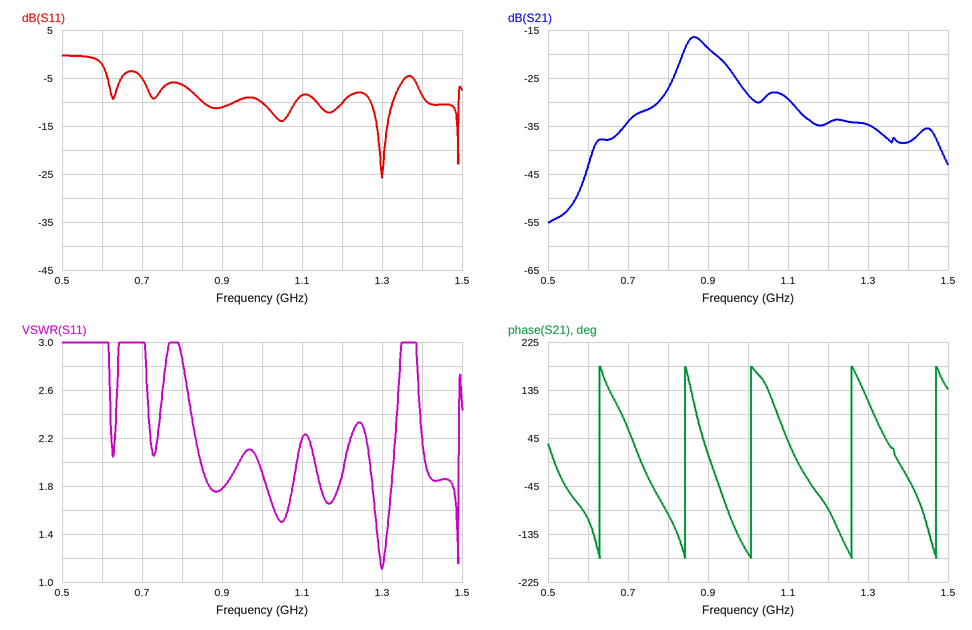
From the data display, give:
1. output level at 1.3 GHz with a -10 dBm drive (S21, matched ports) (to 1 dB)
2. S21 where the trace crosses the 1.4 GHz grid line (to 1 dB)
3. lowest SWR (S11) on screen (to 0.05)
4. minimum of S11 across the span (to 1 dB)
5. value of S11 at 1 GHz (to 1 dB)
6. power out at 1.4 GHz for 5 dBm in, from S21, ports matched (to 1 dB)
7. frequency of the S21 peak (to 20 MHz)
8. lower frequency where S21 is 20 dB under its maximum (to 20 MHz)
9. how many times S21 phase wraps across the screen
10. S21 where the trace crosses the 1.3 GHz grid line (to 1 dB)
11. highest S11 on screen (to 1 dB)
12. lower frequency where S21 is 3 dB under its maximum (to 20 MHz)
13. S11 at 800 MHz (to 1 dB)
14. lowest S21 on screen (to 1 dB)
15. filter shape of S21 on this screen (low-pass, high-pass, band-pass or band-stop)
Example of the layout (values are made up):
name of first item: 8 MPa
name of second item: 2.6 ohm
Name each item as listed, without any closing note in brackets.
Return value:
output level at 1.3 GHz with a -10 dBm drive (S21, matched ports): -45 dBm
S21 where the trace crosses the 1.4 GHz grid line: -38 dB
lowest SWR (S11) on screen: 1.10
minimum of S11 across the span: -26 dB
value of S11 at 1 GHz: -10 dB
power out at 1.4 GHz for 5 dBm in, from S21, ports matched: -33 dBm
frequency of the S21 peak: 860 MHz
lower frequency where S21 is 20 dB under its maximum: 680 MHz
how many times S21 phase wraps across the screen: 5
S21 where the trace crosses the 1.3 GHz grid line: -35 dB
highest S11 on screen: 0 dB
lower frequency where S21 is 3 dB under its maximum: 840 MHz
S11 at 800 MHz: -6 dB
lowest S21 on screen: -55 dB
filter shape of S21 on this screen: band-pass
